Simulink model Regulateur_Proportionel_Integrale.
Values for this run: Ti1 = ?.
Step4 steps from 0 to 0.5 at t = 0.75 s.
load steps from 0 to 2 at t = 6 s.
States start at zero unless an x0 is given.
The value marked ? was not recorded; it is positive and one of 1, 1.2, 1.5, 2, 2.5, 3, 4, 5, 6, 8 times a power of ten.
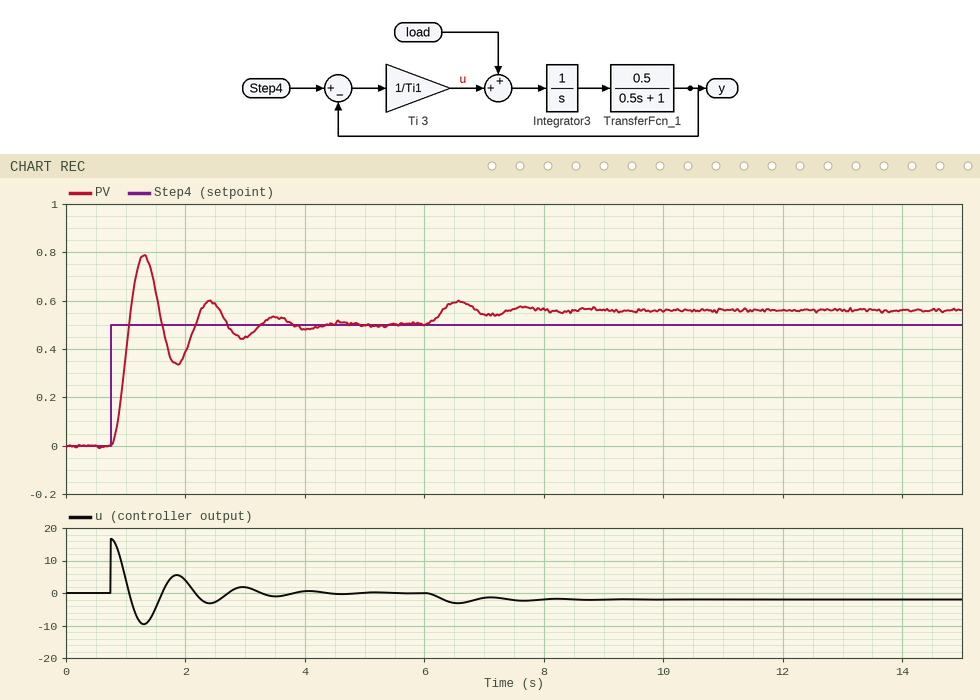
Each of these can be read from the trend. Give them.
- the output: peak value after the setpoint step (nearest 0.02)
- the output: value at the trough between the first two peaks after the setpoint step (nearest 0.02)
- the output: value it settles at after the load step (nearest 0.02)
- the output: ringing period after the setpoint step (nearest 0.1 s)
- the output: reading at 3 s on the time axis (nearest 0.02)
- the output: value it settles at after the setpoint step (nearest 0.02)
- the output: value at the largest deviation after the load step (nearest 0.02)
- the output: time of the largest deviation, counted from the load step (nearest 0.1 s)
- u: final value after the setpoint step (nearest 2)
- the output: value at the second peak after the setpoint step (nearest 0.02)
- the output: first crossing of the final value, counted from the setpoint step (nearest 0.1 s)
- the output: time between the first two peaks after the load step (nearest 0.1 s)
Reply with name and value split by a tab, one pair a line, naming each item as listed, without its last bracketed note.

the output: peak value after the setpoint step	0.78
the output: value at the trough between the first two peaks after the setpoint step	0.34
the output: value it settles at after the load step	0.56
the output: ringing period after the setpoint step	1.1 s
the output: reading at 3 s on the time axis	0.44
the output: value it settles at after the setpoint step	0.50
the output: value at the largest deviation after the load step	0.60
the output: time of the largest deviation, counted from the load step	0.6 s
u: final value after the setpoint step	0
the output: value at the second peak after the setpoint step	0.60
the output: first crossing of the final value, counted from the setpoint step	0.3 s
the output: time between the first two peaks after the load step	1.1 s
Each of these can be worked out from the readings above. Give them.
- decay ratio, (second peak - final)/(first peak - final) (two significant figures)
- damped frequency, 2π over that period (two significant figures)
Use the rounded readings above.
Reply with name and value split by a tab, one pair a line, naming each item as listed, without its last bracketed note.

decay ratio, (second peak - final)/(first peak - final)	0.36
damped frequency, 2π over that period	5.7 rad/s
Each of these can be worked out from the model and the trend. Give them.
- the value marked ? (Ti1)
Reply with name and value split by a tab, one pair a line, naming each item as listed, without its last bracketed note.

the value marked ?	0.03
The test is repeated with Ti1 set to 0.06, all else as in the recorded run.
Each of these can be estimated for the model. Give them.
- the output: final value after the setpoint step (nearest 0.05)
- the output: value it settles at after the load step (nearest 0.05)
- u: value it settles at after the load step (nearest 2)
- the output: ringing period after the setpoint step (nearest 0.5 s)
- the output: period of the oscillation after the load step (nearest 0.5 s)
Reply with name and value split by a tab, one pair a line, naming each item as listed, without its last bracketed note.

the output: final value after the setpoint step	0.50
the output: value it settles at after the load step	0.60
u: value it settles at after the load step	-2
the output: ringing period after the setpoint step	1.5 s
the output: period of the oscillation after the load step	1.5 s
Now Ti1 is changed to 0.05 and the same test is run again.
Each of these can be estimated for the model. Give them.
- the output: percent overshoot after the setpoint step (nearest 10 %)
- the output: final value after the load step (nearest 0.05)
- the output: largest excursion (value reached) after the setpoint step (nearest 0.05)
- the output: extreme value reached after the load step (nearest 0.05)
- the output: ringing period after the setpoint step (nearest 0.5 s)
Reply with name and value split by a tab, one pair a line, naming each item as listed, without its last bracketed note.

the output: percent overshoot after the setpoint step	50 %
the output: final value after the load step	0.60
the output: largest excursion (value reached) after the setpoint step	0.75
the output: extreme value reached after the load step	0.65
the output: ringing period after the setpoint step	1.5 s
